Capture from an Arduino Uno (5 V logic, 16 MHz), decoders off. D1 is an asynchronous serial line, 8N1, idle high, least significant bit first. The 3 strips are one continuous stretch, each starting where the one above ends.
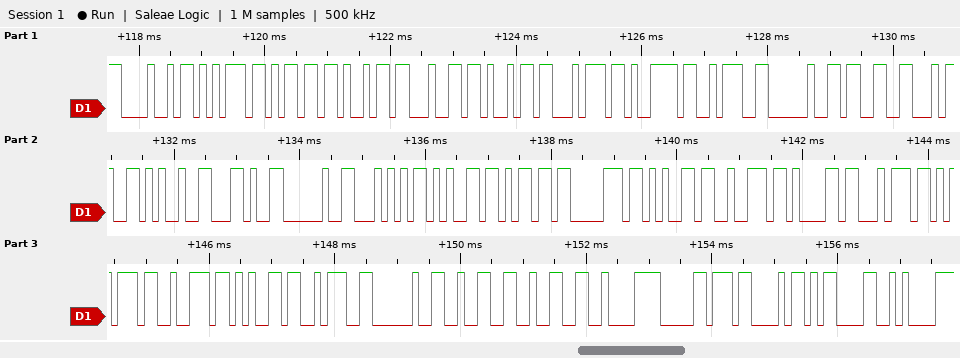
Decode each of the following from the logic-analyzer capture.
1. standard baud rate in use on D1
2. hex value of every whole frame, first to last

9600 baud
48 75 6D 69 64 69 74 79 3A 20 33 34 25 2C 20 54 65 6D 70 65 72 61 74 75 72 65 3A 20 32 32 C2 B0 43 0D 0A
